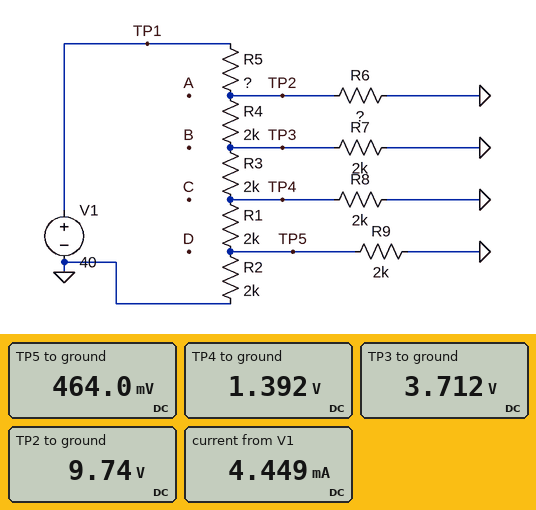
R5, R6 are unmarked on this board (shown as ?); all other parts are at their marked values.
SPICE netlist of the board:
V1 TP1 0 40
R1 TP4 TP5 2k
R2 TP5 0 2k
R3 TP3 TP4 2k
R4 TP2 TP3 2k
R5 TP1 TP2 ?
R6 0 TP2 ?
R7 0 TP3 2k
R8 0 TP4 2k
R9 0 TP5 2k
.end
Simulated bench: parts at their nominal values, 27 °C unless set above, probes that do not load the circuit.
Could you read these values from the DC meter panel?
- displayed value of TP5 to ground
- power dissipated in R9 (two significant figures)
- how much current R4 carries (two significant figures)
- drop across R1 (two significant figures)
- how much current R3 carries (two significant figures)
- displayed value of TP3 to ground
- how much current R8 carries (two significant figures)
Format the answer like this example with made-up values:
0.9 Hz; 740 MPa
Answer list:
464.0 mV; 110 µW; 3.0 mA; 930 mV; 1.2 mA; 3.712 V; 700 µA
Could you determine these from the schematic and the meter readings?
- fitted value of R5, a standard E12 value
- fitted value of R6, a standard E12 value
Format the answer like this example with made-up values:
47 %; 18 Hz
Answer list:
6.8 kΩ; 6.8 kΩ
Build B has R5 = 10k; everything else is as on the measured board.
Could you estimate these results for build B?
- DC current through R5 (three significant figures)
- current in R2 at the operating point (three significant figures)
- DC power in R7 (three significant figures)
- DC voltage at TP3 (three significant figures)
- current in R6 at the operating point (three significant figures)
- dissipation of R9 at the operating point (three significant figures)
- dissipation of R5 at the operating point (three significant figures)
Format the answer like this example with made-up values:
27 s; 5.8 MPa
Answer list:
3.28 mA; 171 µA; 3.75 mW; 2.74 V; 1.06 mA; 58.6 µW; 108 mW
